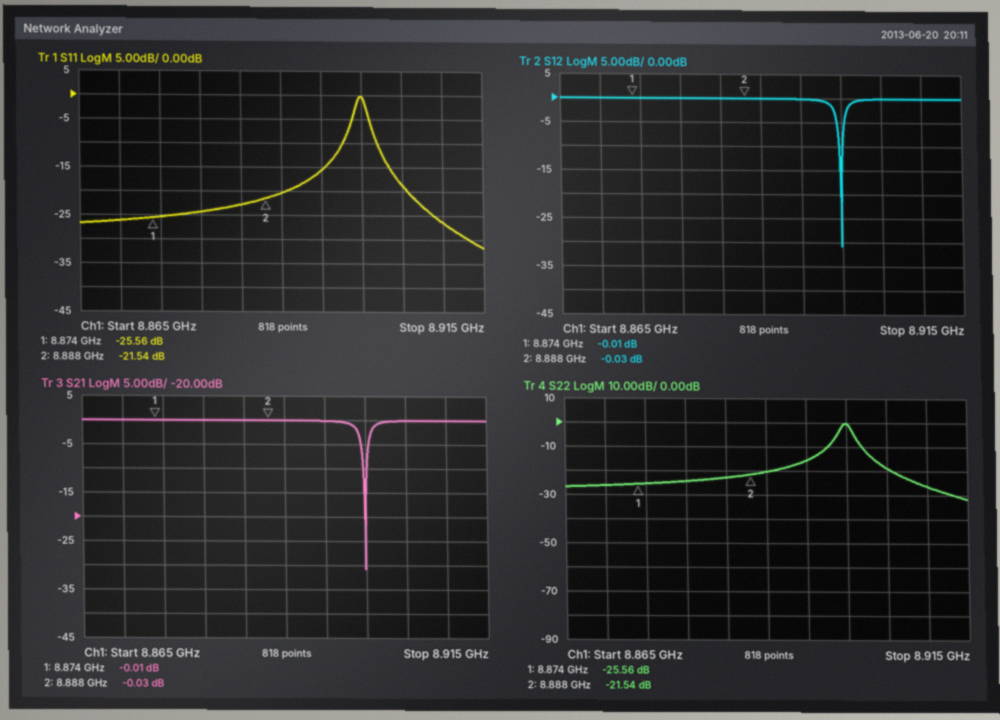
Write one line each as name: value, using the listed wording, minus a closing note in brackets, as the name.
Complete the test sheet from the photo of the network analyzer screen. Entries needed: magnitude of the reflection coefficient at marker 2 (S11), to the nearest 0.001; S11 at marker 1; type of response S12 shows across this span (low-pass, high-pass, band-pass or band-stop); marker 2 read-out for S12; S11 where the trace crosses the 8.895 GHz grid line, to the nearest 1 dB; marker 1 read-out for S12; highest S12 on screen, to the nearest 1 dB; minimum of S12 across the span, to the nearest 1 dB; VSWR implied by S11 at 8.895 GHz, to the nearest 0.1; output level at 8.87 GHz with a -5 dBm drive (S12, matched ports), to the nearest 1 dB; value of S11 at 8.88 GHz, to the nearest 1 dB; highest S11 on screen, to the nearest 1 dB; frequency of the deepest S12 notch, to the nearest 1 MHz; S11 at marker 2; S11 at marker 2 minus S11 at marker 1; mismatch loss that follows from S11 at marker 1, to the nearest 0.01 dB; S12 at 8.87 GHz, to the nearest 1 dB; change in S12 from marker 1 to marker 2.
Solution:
magnitude of the reflection coefficient at marker 2 (S11), to the nearest 0.001: 0.084
S11 at marker 1: -25.56 dB
type of response S12 shows across this span: band-stop
marker 2 read-out for S12: -0.03 dB
S11 where the trace crosses the 8.895 GHz grid line, to the nearest 1 dB: -16 dB
marker 1 read-out for S12: -0.01 dB
highest S12 on screen, to the nearest 1 dB: 0 dB
minimum of S12 across the span, to the nearest 1 dB: -31 dB
VSWR implied by S11 at 8.895 GHz, to the nearest 0.1: 1.4
output level at 8.87 GHz with a -5 dBm drive (S12, matched ports), to the nearest 1 dB: -5 dBm
value of S11 at 8.88 GHz, to the nearest 1 dB: -24 dB
highest S11 on screen, to the nearest 1 dB: 0 dB
frequency of the deepest S12 notch, to the nearest 1 MHz: 8.900 GHz
S11 at marker 2: -21.54 dB
S11 at marker 2 minus S11 at marker 1: 4.02 dB
mismatch loss that follows from S11 at marker 1, to the nearest 0.01 dB: 0.01 dB
S12 at 8.87 GHz, to the nearest 1 dB: 0 dB
change in S12 from marker 1 to marker 2: -0.02 dB
